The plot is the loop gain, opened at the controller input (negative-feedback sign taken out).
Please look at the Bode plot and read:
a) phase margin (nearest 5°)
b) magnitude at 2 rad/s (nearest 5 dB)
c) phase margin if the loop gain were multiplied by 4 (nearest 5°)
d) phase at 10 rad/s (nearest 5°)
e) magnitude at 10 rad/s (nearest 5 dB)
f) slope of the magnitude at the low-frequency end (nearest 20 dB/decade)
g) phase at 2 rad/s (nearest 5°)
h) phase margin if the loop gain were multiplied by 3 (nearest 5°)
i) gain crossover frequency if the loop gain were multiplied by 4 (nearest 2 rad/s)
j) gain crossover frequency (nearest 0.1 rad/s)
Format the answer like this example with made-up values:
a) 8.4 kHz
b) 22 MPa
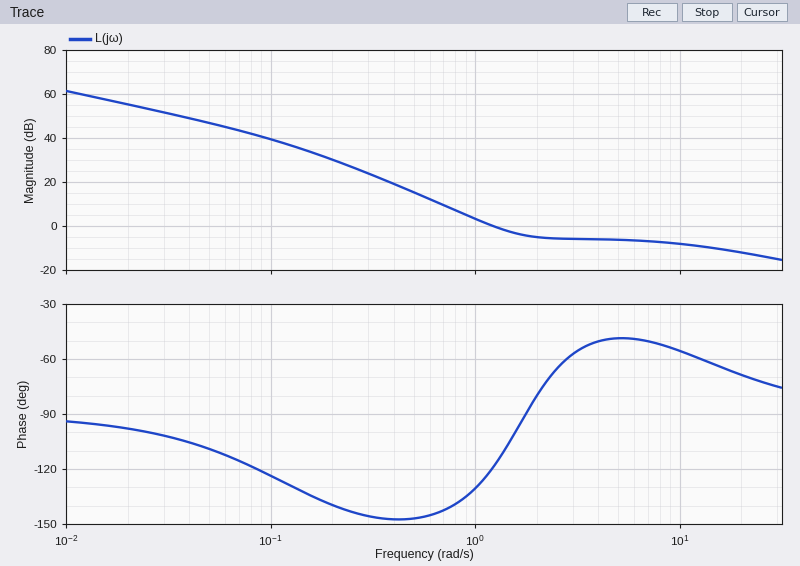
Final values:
a) 60°
b) -5 dB
c) 110°
d) -55°
e) -10 dB
f) -20 dB/decade
g) -80°
h) 120°
i) 20 rad/s
j) 1.2 rad/s
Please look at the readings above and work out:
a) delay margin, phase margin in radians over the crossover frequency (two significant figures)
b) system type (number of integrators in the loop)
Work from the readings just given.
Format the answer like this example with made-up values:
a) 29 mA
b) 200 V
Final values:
a) 0.87 s
b) 1
